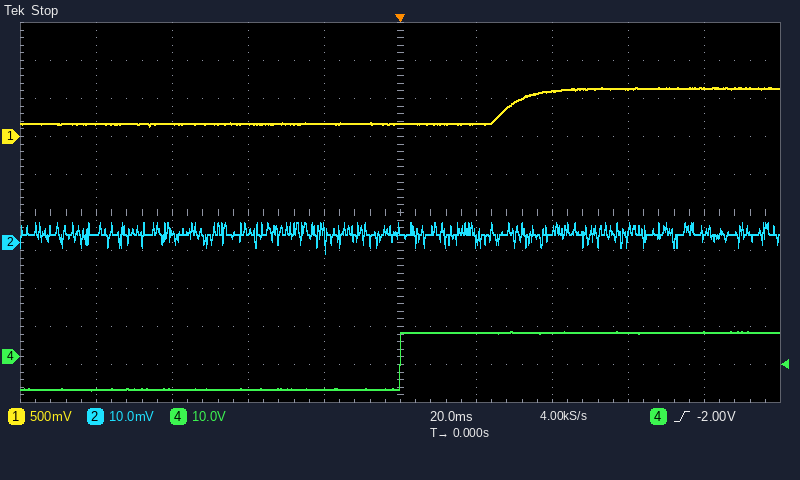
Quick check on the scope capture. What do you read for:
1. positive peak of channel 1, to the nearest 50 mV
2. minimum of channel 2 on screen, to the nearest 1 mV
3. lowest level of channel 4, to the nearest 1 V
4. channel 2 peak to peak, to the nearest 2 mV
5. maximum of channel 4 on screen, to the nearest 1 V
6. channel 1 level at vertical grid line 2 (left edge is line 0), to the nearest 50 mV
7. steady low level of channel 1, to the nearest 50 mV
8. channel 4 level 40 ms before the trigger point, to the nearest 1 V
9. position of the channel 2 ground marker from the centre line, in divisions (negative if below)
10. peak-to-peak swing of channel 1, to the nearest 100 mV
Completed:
650 mV
-3 mV
-9 V
8 mV
7 V
150 mV
150 mV
-9 V
-0.8 div
500 mV
